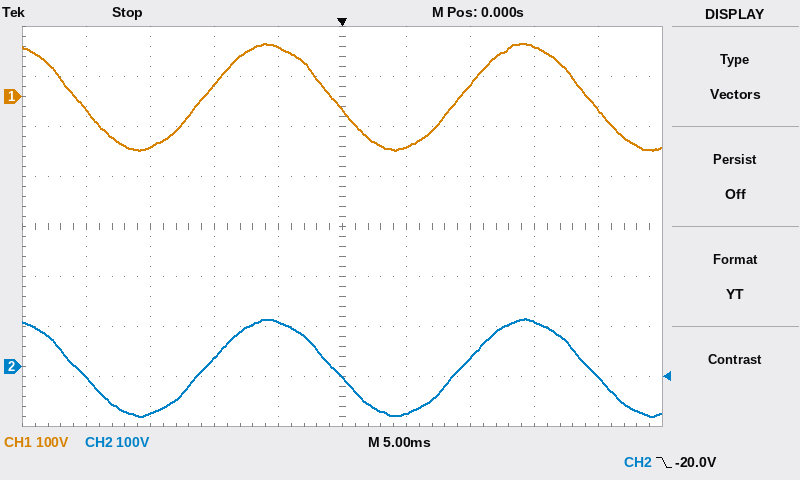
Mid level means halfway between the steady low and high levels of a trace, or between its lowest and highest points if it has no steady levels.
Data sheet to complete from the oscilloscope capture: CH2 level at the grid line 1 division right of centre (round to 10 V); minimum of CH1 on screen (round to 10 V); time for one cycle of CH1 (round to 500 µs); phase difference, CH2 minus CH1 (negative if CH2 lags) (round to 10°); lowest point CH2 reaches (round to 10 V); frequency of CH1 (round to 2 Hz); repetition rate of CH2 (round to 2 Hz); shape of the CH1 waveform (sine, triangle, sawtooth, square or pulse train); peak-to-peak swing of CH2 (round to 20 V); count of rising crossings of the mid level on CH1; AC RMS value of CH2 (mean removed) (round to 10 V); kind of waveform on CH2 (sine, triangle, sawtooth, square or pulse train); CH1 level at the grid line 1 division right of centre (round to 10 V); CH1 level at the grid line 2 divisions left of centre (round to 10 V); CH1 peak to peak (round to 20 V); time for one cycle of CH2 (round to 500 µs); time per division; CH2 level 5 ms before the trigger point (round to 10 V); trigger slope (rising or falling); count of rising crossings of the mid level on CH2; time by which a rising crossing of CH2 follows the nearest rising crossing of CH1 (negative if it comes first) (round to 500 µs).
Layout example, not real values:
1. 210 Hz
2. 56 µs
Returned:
1. -90 V
2. -110 V
3. 20.0 ms
4. 0°
5. -100 V
6. 50 Hz
7. 50 Hz
8. sine
9. 200 V
10. 2
11. 70 V
12. sine
13. -100 V
14. 20 V
15. 220 V
16. 20.0 ms
17. 5 ms
18. 90 V
19. falling
20. 2
21. 0.0 ms
